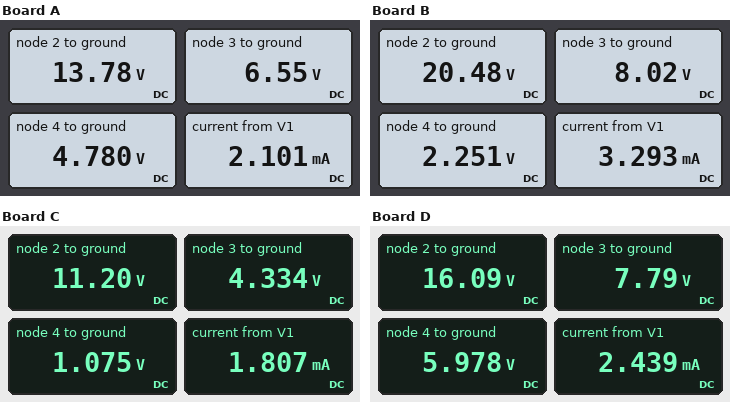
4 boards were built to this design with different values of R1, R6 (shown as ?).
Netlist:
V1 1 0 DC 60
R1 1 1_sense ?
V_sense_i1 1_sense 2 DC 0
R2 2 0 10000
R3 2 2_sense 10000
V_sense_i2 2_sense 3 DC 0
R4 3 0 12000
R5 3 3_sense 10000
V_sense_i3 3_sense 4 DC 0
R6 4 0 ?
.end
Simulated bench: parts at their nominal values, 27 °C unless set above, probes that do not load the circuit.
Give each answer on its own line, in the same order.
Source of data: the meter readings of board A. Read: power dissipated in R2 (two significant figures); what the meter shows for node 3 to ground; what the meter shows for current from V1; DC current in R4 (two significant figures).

19 mW
6.55 V
2.101 mA
550 µA
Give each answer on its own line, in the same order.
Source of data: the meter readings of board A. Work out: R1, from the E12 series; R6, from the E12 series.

22 kΩ
27 kΩ
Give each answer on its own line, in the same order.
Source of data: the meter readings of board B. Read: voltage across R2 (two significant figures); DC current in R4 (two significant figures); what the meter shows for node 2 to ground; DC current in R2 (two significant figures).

20 V
670 µA
20.48 V
2.0 mA
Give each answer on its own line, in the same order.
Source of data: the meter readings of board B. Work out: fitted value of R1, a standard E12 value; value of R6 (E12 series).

12 kΩ
3.9 kΩ
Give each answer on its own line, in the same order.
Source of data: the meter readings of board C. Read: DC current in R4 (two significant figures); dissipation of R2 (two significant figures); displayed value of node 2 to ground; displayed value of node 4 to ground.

360 µA
13 mW
11.20 V
1.075 V
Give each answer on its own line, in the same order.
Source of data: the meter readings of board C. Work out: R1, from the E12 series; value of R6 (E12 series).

27 kΩ
3.3 kΩ
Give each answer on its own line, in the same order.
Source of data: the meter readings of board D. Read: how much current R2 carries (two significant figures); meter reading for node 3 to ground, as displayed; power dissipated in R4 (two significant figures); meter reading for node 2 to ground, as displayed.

1.6 mA
7.79 V
5.1 mW
16.09 V
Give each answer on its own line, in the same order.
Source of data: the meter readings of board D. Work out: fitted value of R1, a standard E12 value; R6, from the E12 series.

18 kΩ
33 kΩ
